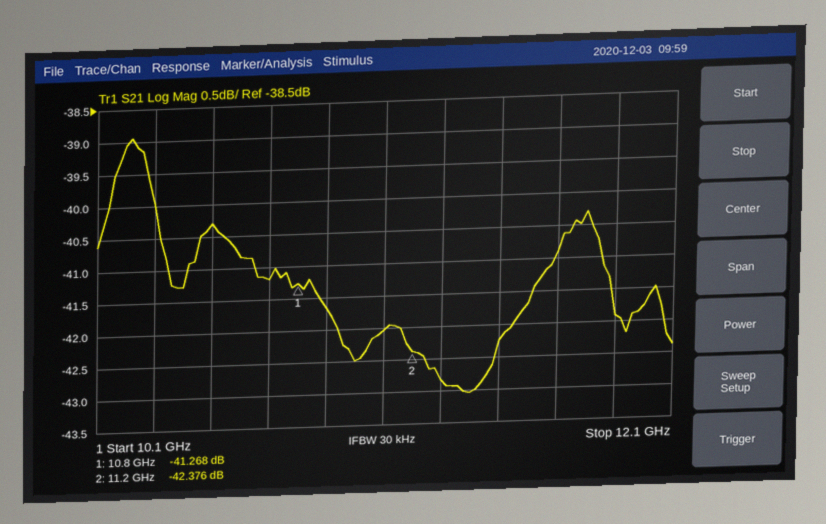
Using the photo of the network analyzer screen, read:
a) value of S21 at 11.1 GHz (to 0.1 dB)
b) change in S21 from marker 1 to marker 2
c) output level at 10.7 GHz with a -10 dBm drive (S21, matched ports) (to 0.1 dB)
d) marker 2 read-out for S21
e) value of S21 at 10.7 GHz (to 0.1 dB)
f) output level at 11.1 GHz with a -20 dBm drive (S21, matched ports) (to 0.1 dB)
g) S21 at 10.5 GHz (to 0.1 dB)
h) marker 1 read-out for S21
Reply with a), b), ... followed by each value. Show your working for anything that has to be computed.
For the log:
a) -42.0 dB
b) -42.376 − (-41.268) = -1.108 dB
c) -10 dBm + (-41.2 dB) = -51.2 dBm
d) -42.376 dB
e) -41.2 dB
f) -20 dBm + (-42.0 dB) = -62.0 dBm
g) -40.3 dB
h) -41.268 dB
